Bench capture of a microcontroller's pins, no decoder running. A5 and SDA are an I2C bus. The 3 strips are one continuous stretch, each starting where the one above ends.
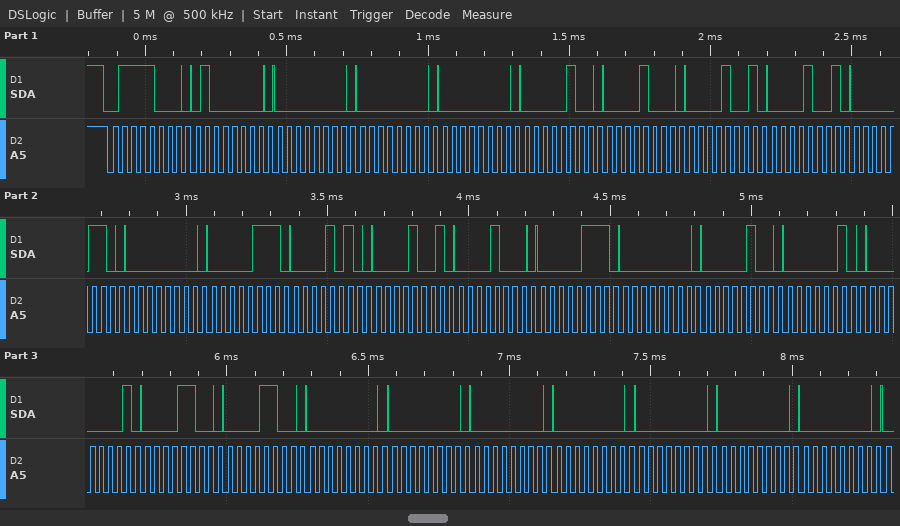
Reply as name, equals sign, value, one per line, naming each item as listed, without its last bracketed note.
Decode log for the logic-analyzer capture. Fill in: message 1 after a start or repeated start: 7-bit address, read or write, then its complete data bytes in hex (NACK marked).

message 1 after a start or repeated start: 7-bit address, read or write, then its complete data bytes in hex = 0x3C write: 40 00 00 00 04 08 09 09 06 00 07 0A 09 08 07 00 04 02 01 0C 0C 00 00 00 00 00 00 00
